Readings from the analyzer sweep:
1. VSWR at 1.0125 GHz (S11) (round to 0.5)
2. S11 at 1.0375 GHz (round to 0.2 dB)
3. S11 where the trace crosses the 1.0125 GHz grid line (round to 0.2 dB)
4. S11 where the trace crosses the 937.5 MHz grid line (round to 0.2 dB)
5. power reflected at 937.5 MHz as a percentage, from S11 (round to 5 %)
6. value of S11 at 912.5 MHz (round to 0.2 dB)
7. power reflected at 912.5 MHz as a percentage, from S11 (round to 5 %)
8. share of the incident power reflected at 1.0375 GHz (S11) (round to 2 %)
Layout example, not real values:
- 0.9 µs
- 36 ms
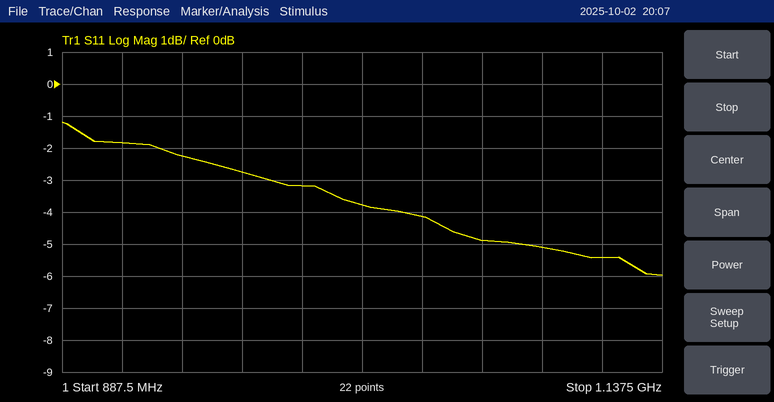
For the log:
- 4.5
- -4.2 dB
- -3.8 dB
- -2.2 dB
- 60 %
- -1.8 dB
- 65 %
- 38 %
